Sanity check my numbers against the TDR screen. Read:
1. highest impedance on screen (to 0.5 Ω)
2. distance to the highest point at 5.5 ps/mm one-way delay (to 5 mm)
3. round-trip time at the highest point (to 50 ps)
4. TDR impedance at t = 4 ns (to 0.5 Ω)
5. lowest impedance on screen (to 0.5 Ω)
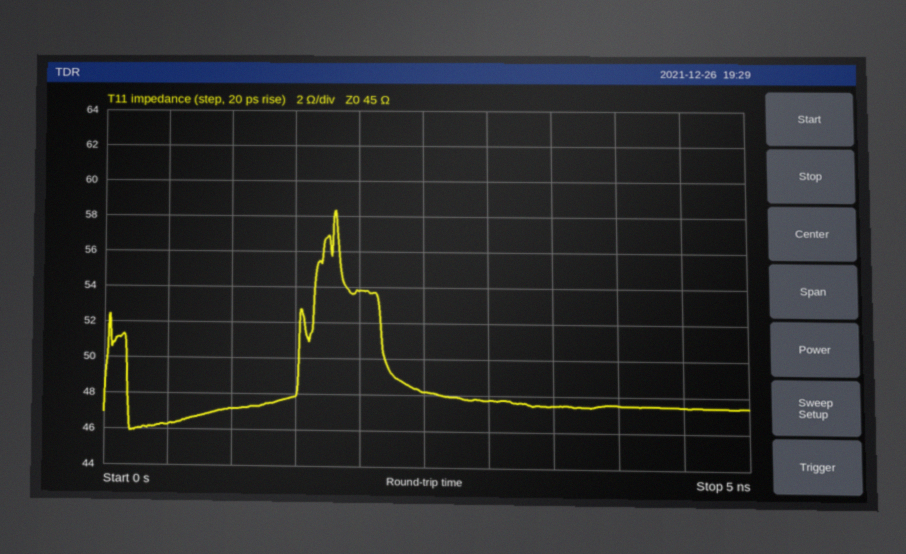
58.5 Ω
165 mm
1.80 ns
47.5 Ω
46.0 Ω
